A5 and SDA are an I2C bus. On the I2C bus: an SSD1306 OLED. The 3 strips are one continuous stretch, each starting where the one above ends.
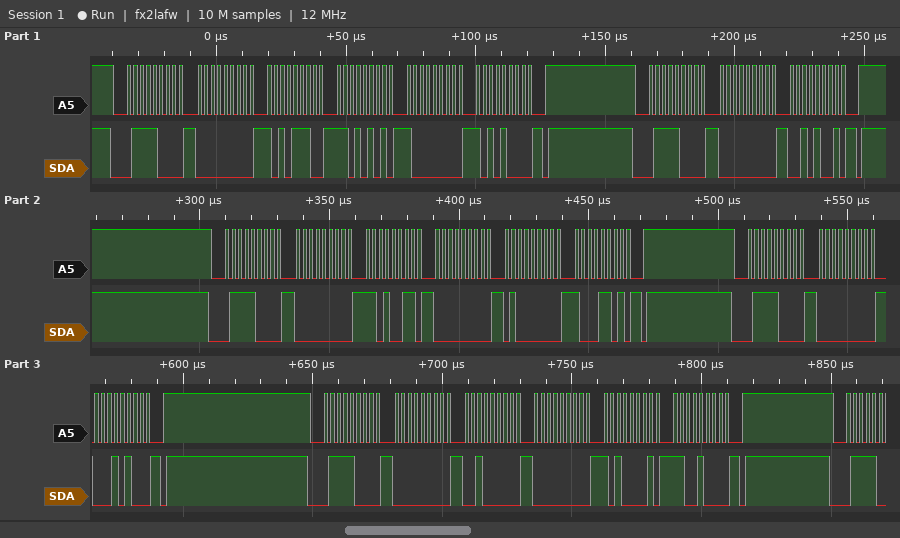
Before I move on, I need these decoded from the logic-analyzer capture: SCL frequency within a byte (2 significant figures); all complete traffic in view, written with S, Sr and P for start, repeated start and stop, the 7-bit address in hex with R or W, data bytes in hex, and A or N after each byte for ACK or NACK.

400 kHz
S 3CW A 00 A AE A D5 A 80 A A8 A P S 3CW A 00 A 29 A P S 3CW A 00 A D3 A 00 A 40 A 8D A P S 3CW A 00 A 14 A P S 3CW A 00 A 20 A 00 A A1 A C8 A P
